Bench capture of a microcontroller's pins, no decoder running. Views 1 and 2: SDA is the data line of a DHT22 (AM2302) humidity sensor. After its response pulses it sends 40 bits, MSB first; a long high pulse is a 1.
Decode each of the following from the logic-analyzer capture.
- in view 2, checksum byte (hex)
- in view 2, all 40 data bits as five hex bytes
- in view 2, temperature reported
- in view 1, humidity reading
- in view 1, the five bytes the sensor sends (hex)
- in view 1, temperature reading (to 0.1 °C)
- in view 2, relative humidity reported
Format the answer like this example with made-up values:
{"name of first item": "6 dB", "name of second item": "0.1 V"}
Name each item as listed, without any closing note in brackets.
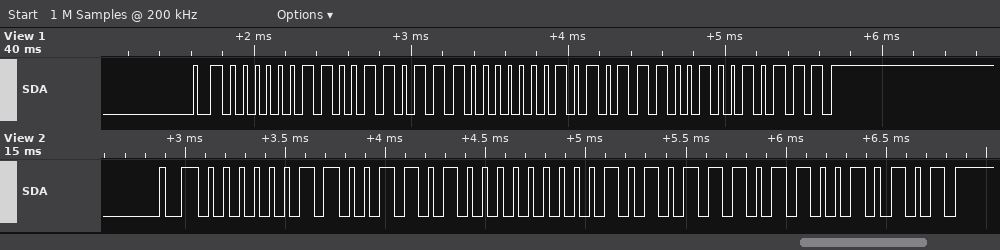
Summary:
{"in view 2, checksum byte": "0x95", "in view 2, all 40 data bits as five hex bytes": "03 34 01 5D 95", "in view 2, temperature reported": "34.9 °C", "in view 1, humidity reading": "82.3 %", "in view 1, the five bytes the sensor sends": "03 37 01 5C 97", "in view 1, temperature reading": "34.8 °C", "in view 2, relative humidity reported": "82.0 %"}
